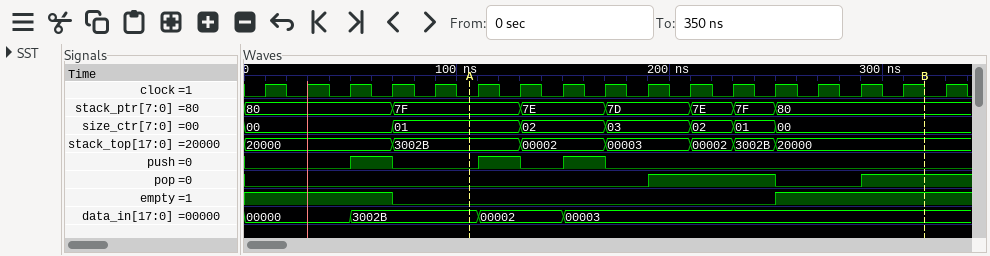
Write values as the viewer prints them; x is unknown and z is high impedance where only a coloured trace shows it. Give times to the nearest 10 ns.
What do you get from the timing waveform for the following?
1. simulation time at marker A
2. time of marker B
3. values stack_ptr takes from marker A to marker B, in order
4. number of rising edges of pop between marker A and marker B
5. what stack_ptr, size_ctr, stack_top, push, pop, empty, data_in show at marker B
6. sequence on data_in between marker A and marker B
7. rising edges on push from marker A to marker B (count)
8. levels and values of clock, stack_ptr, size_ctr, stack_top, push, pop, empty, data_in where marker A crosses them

110 ns
320 ns
7F, 7E, 7D, 7E, 7F, 80
2
stack_ptr=80, size_ctr=00, stack_top=20000, push=0, pop=1, empty=1, data_in=00003
3002B, 00002, 00003
2
clock=0, stack_ptr=7F, size_ctr=01, stack_top=3002B, push=0, pop=0, empty=0, data_in=3002B
